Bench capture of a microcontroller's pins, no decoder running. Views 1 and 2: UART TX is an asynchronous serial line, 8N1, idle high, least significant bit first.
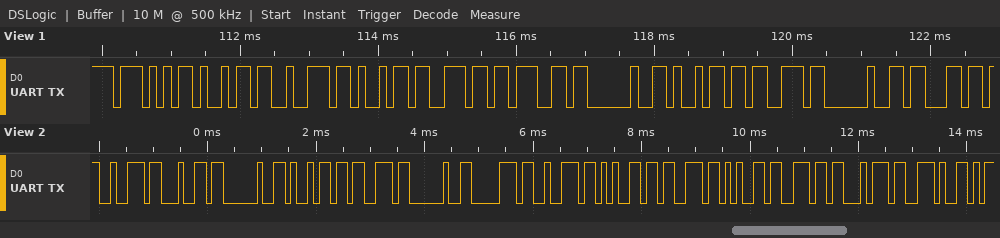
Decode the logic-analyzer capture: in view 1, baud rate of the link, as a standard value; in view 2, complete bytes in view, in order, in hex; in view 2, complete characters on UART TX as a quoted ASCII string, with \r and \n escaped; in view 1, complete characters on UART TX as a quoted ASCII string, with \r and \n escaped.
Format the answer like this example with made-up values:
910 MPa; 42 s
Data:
9600 baud; 72 64 20 69 73 20 70 72 65 73 65 6E 74 2E; "rd is present."; "Wiring is c"
